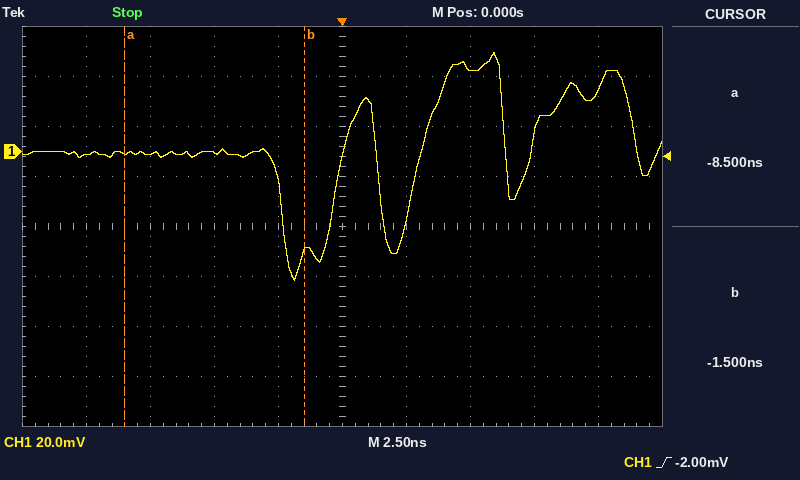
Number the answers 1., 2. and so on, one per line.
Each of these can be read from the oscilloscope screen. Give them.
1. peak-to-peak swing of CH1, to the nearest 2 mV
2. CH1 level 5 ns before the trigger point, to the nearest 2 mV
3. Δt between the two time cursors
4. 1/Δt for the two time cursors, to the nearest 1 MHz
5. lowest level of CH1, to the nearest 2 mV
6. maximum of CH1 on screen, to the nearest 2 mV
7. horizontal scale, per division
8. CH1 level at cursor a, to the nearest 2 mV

1. 92 mV
2. 0 mV
3. 7.00 ns
4. 143 MHz
5. -52 mV
6. 40 mV
7. 2.5 ns
8. 0 mV
